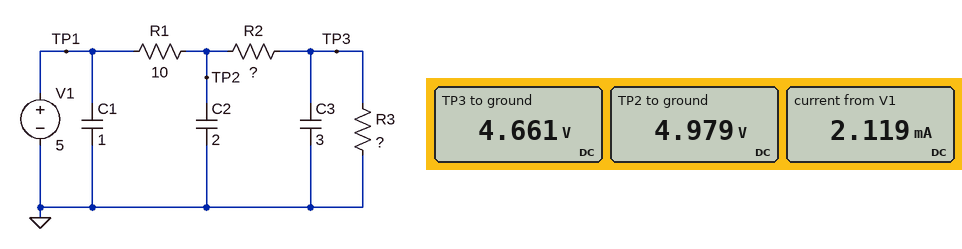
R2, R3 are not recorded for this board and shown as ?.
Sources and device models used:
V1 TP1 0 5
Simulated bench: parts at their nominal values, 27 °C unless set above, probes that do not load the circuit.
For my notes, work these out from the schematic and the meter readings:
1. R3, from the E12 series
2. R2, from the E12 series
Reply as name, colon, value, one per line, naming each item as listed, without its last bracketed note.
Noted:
R3, from the E12 series: 2.2 kΩ
R2, from the E12 series: 150 Ω
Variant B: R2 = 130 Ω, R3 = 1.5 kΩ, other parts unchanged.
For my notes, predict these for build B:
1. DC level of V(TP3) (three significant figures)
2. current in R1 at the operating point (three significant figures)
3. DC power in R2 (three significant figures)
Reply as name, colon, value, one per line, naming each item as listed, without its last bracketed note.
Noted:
DC level of V(TP3): 4.57 V
current in R1 at the operating point: 3.05 mA
DC power in R2: 1.21 mW
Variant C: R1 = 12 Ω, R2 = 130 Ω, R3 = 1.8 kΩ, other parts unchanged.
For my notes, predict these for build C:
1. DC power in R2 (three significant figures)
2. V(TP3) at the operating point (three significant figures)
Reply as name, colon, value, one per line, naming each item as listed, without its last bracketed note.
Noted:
DC power in R2: 862 µW
V(TP3) at the operating point: 4.63 V
